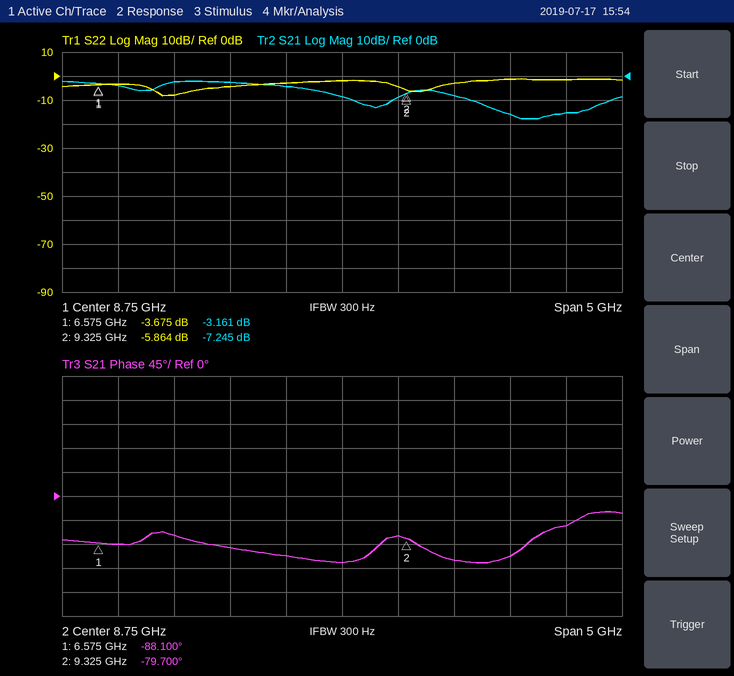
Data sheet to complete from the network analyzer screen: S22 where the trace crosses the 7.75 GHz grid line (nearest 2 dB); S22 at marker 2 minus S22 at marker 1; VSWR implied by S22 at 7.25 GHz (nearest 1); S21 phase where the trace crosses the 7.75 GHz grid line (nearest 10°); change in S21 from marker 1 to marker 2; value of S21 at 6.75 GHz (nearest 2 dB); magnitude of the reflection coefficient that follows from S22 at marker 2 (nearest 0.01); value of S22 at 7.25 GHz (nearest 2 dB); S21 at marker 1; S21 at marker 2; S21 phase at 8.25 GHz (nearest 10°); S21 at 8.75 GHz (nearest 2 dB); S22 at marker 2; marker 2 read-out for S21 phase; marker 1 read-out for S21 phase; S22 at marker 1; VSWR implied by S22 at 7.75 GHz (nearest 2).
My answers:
-4 dB
-2.189 dB
2
-100°
-4.084 dB
-4 dB
0.51
-8 dB
-3.161 dB
-7.245 dB
-110°
-8 dB
-5.864 dB
-79.700°
-88.100°
-3.675 dB
4
